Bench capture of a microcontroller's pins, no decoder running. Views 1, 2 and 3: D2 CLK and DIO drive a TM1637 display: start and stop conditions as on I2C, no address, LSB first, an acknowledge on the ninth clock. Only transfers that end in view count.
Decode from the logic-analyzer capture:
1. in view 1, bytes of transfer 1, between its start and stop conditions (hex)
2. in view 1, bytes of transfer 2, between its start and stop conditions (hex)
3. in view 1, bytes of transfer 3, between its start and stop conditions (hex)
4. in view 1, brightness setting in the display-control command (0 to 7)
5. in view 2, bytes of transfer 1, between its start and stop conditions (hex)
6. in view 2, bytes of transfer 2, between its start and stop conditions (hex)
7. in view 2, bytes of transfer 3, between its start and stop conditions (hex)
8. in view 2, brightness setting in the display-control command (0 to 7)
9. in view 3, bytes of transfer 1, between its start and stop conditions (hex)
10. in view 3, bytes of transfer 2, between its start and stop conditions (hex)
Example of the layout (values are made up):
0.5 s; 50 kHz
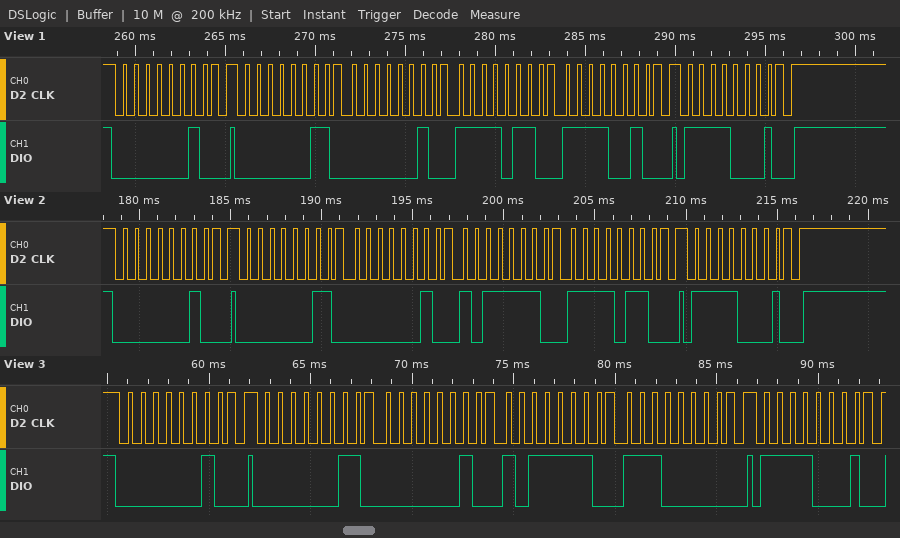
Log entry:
40; C0 40 6F 4F; 8F; 7; 40; C0 40 7D 6F; 8F; 7; 40; C0 40 7D 07
